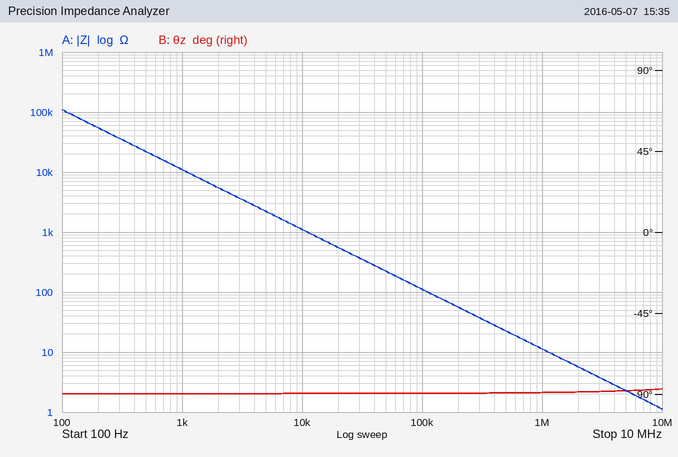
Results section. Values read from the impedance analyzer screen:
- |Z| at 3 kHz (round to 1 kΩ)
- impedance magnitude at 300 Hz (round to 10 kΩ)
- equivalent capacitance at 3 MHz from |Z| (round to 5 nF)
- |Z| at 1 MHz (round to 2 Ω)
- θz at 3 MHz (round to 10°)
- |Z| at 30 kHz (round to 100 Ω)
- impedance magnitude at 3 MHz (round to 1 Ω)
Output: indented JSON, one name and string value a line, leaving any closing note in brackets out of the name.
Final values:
{
  "|Z| at 3 kHz": "4 kΩ",
  "impedance magnitude at 300 Hz": "40 kΩ",
  "equivalent capacitance at 3 MHz from |Z|": "15 nF",
  "|Z| at 1 MHz": "12 Ω",
  "θz at 3 MHz": "-90°",
  "|Z| at 30 kHz": "400 Ω",
  "impedance magnitude at 3 MHz": "4 Ω"
}
